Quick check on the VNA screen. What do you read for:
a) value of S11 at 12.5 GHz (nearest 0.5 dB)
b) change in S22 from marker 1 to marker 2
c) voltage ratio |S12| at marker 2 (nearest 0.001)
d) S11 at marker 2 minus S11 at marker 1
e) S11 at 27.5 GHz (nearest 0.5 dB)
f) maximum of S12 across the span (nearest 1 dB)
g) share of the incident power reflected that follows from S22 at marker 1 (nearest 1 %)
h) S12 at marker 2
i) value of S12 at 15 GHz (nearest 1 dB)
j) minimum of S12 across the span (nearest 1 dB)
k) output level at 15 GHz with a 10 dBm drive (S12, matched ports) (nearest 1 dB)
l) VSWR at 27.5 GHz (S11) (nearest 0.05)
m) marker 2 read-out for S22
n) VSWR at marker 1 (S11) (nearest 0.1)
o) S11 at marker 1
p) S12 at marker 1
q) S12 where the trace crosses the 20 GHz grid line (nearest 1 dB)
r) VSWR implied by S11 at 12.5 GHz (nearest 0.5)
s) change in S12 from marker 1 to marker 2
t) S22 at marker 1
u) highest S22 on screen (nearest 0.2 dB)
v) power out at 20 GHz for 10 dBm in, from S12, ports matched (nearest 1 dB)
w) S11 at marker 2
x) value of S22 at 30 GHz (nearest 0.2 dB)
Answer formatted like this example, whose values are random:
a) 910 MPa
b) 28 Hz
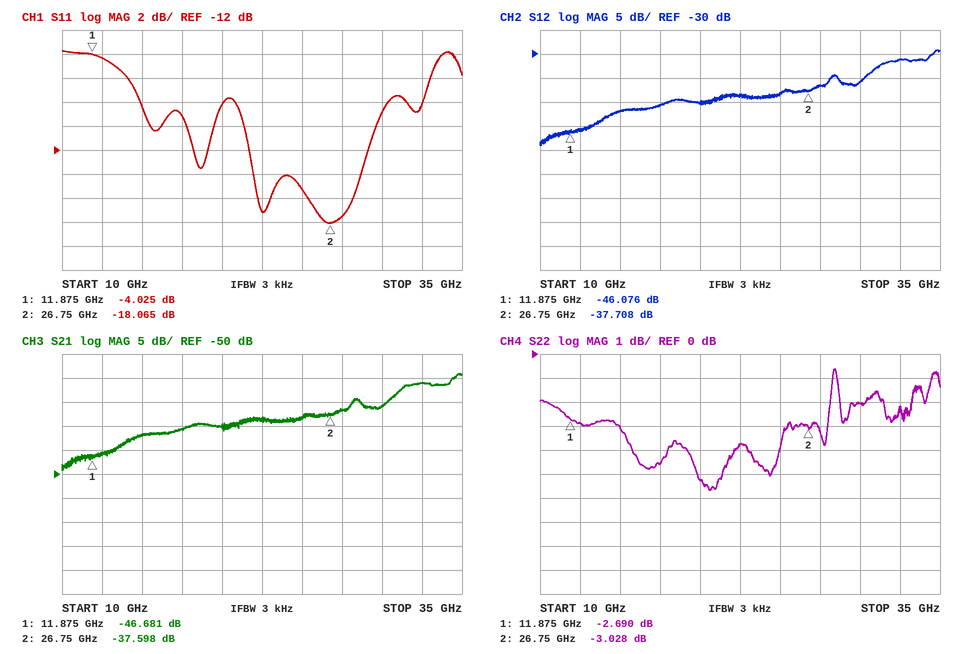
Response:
a) -4.5 dB
b) -0.338 dB
c) 0.013
d) -14.040 dB
e) -17.5 dB
f) -29 dB
g) 54 %
h) -37.708 dB
i) -42 dB
j) -49 dB
k) -32 dBm
l) 1.30
m) -3.028 dB
n) 4.4
o) -4.025 dB
p) -46.076 dB
q) -40 dB
r) 4.0
s) 8.368 dB
t) -2.690 dB
u) -0.6 dB
v) -30 dBm
w) -18.065 dB
x) -2.0 dB
